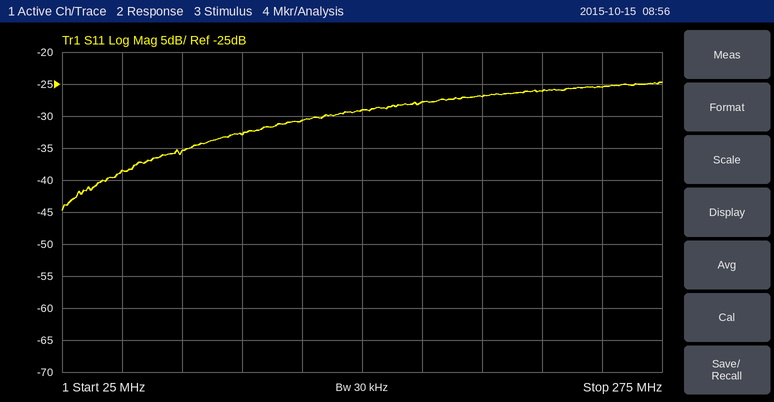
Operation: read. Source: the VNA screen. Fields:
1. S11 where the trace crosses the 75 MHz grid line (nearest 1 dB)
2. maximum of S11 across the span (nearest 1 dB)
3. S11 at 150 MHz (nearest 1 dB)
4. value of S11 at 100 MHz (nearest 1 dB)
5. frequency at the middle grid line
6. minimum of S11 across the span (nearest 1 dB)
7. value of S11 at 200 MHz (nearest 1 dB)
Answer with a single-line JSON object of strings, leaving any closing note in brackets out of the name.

{"S11 where the trace crosses the 75 MHz grid line": "-35 dB", "maximum of S11 across the span": "-25 dB", "S11 at 150 MHz": "-29 dB", "value of S11 at 100 MHz": "-33 dB", "frequency at the middle grid line": "150 MHz", "minimum of S11 across the span": "-45 dB", "value of S11 at 200 MHz": "-27 dB"}
